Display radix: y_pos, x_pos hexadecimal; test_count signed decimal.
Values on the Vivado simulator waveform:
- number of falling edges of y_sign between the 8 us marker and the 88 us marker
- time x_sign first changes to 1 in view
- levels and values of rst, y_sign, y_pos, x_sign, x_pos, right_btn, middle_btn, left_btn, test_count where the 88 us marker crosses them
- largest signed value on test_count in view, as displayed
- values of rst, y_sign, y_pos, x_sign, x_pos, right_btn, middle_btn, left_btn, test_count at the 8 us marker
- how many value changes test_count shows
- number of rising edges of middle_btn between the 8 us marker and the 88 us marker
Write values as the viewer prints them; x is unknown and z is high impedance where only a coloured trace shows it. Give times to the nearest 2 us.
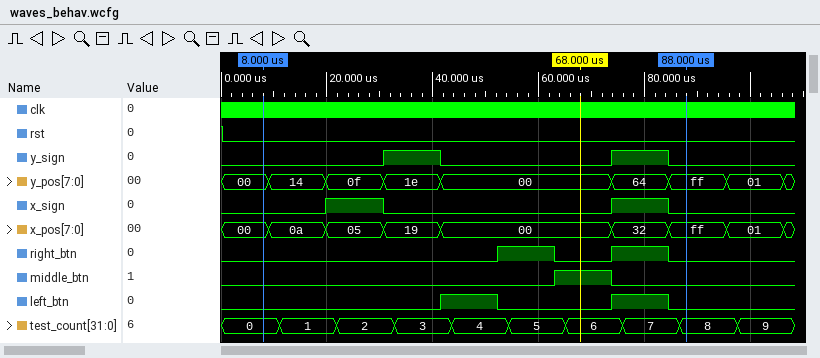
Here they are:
2
20 us
rst=0, y_sign=0, y_pos=ff, x_sign=0, x_pos=ff, right_btn=0, middle_btn=0, left_btn=0, test_count=8
9
rst=0, y_sign=0, y_pos=00, x_sign=0, x_pos=00, right_btn=0, middle_btn=0, left_btn=0, test_count=0
9
1
